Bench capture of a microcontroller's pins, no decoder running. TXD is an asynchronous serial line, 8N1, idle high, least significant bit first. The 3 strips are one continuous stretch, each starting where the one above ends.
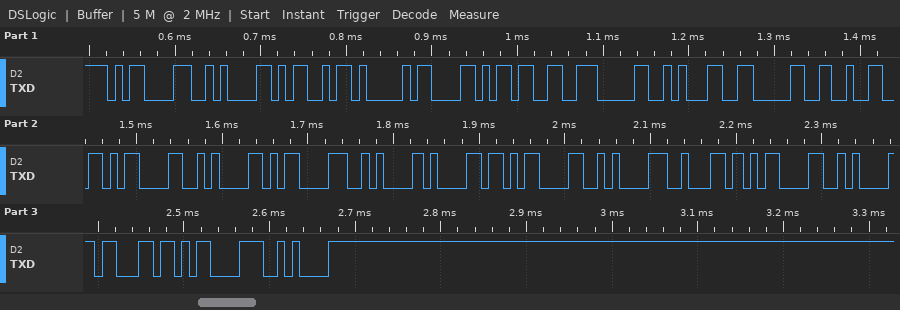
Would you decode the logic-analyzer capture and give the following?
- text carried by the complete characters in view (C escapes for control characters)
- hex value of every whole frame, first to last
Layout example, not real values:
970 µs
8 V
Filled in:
"\r\nMAX30102\r\n\r\na\r\nb\r\nc\r\n"
0D 0A 4D 41 58 33 30 31 30 32 0D 0A 0D 0A 61 0D 0A 62 0D 0A 63 0D 0A
